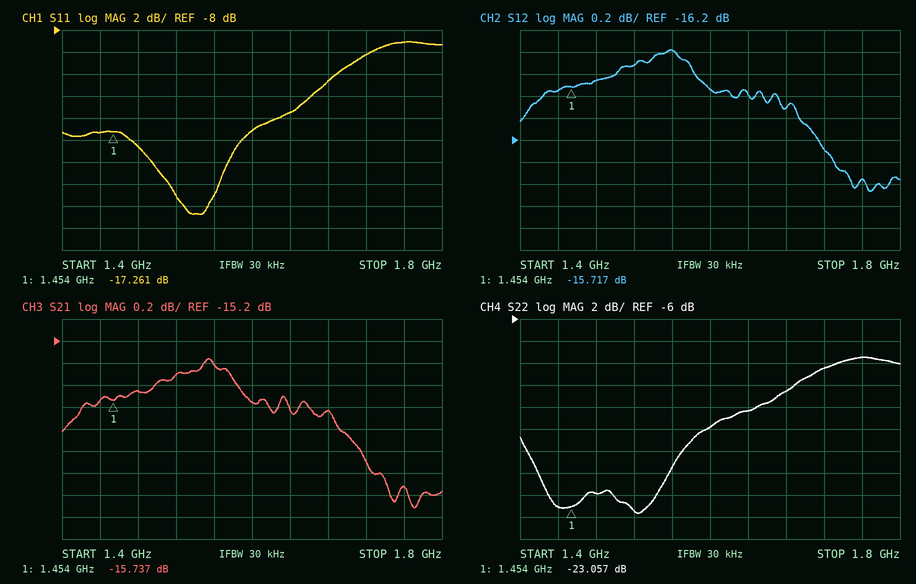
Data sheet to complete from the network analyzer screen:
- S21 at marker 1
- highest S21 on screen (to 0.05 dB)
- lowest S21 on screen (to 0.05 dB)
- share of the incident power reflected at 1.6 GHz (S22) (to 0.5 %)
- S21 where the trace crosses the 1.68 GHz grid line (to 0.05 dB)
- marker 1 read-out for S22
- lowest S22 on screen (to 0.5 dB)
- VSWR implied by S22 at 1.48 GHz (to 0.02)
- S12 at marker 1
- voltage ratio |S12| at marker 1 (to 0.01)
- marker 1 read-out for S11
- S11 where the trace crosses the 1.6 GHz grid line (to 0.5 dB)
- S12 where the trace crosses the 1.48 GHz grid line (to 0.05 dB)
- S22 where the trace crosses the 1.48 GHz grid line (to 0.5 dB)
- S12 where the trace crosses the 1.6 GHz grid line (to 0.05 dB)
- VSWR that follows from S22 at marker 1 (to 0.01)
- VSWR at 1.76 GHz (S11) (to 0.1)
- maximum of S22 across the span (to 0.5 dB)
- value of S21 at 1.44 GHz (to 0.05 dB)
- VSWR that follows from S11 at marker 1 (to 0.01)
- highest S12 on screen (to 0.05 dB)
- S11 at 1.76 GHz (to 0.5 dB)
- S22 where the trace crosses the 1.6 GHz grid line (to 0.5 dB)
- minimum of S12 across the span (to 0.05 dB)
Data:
-15.737 dB
-15.35 dB
-16.70 dB
2.5 %
-15.85 dB
-23.057 dB
-23.5 dB
1.18
-15.717 dB
0.16
-17.261 dB
-17.0 dB
-15.65 dB
-22.0 dB
-15.75 dB
1.15
2.1
-9.5 dB
-15.75 dB
1.32
-15.40 dB
-9.0 dB
-16.0 dB
-16.65 dB
